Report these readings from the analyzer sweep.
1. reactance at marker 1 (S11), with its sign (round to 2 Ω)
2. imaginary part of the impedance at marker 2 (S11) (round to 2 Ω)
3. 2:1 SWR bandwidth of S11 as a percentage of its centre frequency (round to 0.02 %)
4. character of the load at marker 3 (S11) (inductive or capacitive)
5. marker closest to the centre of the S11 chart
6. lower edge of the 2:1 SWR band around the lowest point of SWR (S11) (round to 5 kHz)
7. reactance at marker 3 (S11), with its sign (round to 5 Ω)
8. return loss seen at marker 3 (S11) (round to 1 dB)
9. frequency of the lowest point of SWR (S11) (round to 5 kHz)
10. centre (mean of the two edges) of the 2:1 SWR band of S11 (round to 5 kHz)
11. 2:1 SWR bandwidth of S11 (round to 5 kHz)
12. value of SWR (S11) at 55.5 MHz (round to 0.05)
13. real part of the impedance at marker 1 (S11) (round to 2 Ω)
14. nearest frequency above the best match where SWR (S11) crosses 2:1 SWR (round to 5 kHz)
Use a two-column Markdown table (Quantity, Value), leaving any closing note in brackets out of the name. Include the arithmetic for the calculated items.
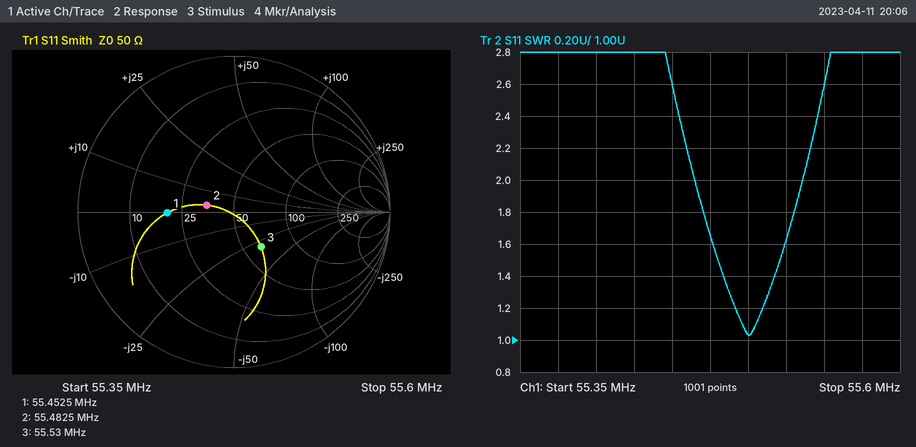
| Quantity | Value |
|---|---|
| reactance at marker 1 (S11), with its sign | 0 Ω |
| imaginary part of the impedance at marker 2 (S11) | +4 Ω |
| 2:1 SWR bandwidth of S11 as a percentage of its centre frequency | 70 kHz / 55.5 MHz ≈ 0.126 %, so 0.12 % to the nearest 0.02 % |
| character of the load at marker 3 (S11) | capacitive |
| marker closest to the centre of the S11 chart | marker 2 |
| lower edge of the 2:1 SWR band around the lowest point of SWR (S11) | 55.465 MHz |
| reactance at marker 3 (S11), with its sign | -30 Ω |
| return loss seen at marker 3 (S11) | 11 dB |
| frequency of the lowest point of SWR (S11) | 55.500 MHz |
| centre (mean of the two edges) of the 2:1 SWR band of S11 | 55.500 MHz |
| 2:1 SWR bandwidth of S11 | 55.535 MHz − 55.465 MHz = 70 kHz |
| value of SWR (S11) at 55.5 MHz | 1.05 |
| real part of the impedance at marker 1 (S11) | 20 Ω |
| nearest frequency above the best match where SWR (S11) crosses 2:1 SWR | 55.535 MHz |
